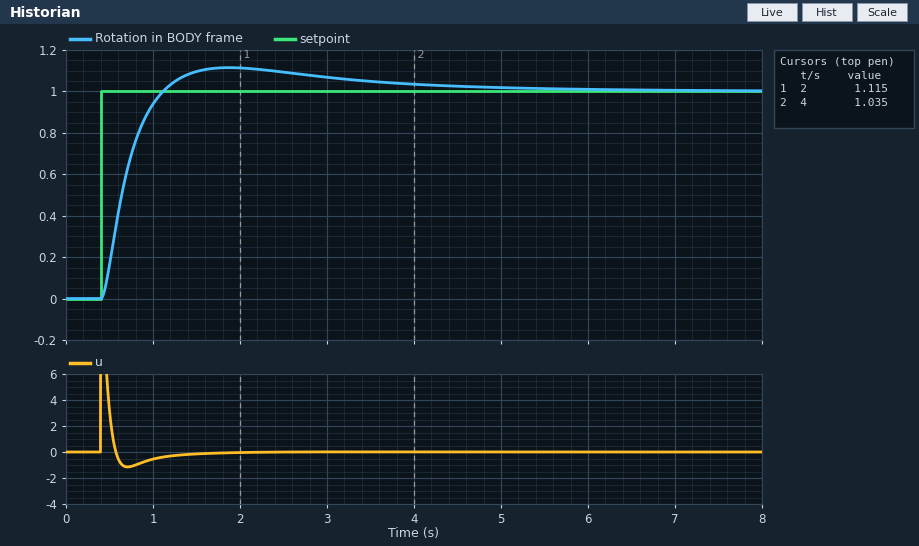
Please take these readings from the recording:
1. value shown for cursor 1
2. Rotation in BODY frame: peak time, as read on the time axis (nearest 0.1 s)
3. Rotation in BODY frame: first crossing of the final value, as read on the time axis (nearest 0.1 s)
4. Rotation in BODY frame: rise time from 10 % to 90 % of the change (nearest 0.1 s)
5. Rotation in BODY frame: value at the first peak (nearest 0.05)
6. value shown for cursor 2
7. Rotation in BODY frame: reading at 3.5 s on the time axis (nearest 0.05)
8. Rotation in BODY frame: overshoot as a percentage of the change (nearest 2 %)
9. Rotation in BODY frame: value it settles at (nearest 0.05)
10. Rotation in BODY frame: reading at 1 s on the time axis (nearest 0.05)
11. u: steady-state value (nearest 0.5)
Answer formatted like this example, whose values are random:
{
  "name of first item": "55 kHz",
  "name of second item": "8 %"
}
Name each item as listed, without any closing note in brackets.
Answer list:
{
  "value shown for cursor 1": "1.115",
  "Rotation in BODY frame: peak time, as read on the time axis": "1.9 s",
  "Rotation in BODY frame: first crossing of the final value, as read on the time axis": "1.1 s",
  "Rotation in BODY frame: rise time from 10 % to 90 % of the change": "0.5 s",
  "Rotation in BODY frame: value at the first peak": "1.10",
  "value shown for cursor 2": "1.035",
  "Rotation in BODY frame: reading at 3.5 s on the time axis": "1.05",
  "Rotation in BODY frame: overshoot as a percentage of the change": "12 %",
  "Rotation in BODY frame: value it settles at": "1.00",
  "Rotation in BODY frame: reading at 1 s on the time axis": "0.95",
  "u: steady-state value": "0.0"
}
